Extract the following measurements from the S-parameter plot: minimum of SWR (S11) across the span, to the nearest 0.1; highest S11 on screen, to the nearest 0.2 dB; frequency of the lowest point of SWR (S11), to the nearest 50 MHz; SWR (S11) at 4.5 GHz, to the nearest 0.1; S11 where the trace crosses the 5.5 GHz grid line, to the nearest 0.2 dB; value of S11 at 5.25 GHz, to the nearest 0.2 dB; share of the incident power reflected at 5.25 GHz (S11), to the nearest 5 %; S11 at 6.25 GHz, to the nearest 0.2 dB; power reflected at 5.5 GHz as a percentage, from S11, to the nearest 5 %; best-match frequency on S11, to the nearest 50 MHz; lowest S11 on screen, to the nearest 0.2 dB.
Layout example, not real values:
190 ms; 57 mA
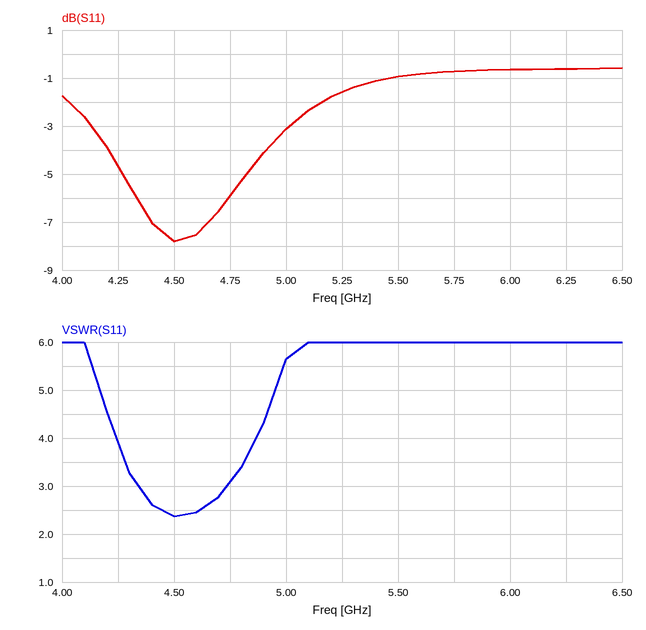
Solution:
2.4; -0.6 dB; 4.50 GHz; 2.4; -1.0 dB; -1.6 dB; 70 %; -0.6 dB; 80 %; 4.50 GHz; -7.8 dB
